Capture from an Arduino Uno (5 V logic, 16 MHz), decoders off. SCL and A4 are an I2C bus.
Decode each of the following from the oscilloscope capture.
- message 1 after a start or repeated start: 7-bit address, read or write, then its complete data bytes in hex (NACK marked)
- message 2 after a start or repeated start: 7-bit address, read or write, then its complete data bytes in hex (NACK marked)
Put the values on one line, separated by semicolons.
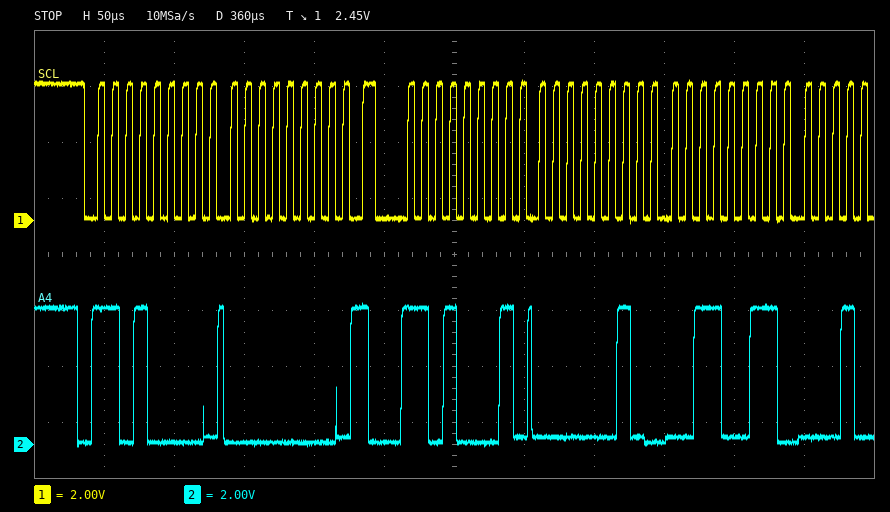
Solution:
0x68 write: 00; 0x68 read: 02 33
